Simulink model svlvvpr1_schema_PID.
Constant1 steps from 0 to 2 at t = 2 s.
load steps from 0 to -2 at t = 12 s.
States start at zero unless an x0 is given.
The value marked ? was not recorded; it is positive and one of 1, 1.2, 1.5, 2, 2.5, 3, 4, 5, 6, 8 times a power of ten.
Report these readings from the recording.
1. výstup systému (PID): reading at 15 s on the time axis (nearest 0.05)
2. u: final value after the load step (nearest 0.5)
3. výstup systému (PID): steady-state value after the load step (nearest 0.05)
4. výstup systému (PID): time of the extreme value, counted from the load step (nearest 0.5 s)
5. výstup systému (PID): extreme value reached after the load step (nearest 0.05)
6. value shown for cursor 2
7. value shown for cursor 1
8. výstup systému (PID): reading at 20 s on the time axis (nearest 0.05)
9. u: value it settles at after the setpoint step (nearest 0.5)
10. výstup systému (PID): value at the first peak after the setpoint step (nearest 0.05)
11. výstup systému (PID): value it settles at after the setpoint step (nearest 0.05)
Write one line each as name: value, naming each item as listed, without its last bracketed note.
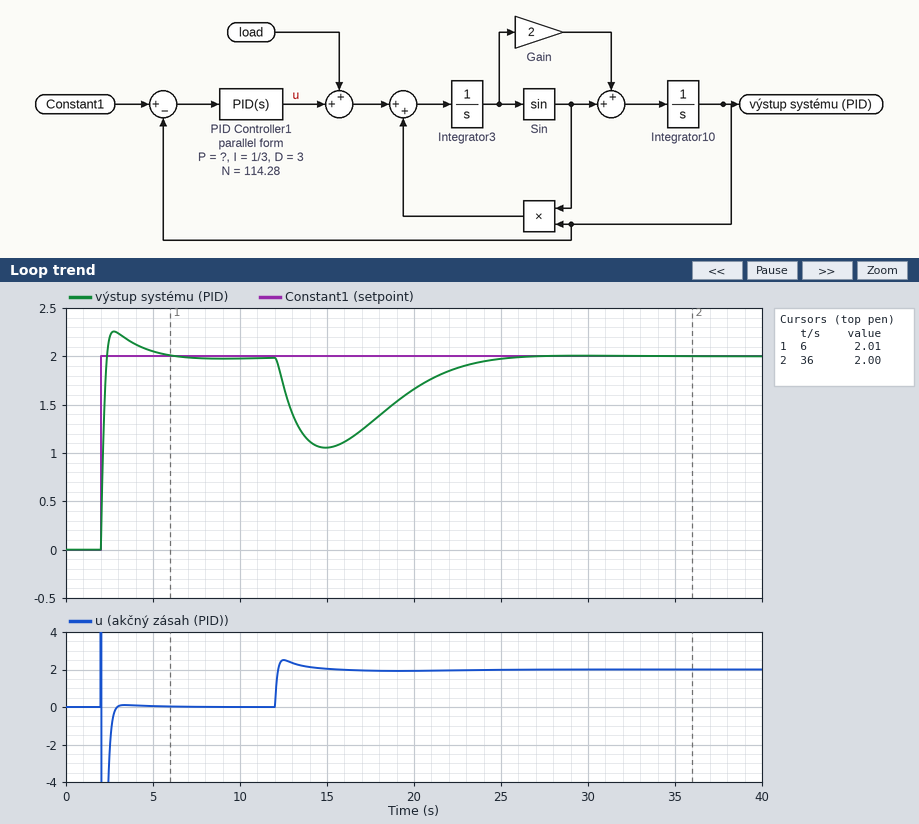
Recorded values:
výstup systému (PID): reading at 15 s on the time axis: 1.05
u: final value after the load step: 2.0
výstup systému (PID): steady-state value after the load step: 2.00
výstup systému (PID): time of the extreme value, counted from the load step: 3.0 s
výstup systému (PID): extreme value reached after the load step: 1.05
value shown for cursor 2: 2.00
value shown for cursor 1: 2.01
výstup systému (PID): reading at 20 s on the time axis: 1.65
u: value it settles at after the setpoint step: 0.0
výstup systému (PID): value at the first peak after the setpoint step: 2.25
výstup systému (PID): value it settles at after the setpoint step: 2.00
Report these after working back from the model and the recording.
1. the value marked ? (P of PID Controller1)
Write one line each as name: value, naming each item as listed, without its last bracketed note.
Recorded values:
the value marked ?: 1.5
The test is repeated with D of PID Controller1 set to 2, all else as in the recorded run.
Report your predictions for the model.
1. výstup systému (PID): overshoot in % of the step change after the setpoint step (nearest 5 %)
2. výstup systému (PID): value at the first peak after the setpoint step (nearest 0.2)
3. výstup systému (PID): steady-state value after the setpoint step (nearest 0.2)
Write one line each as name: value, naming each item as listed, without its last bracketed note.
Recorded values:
výstup systému (PID): overshoot in % of the step change after the setpoint step: 25 %
výstup systému (PID): value at the first peak after the setpoint step: 2.6
výstup systému (PID): steady-state value after the setpoint step: 2.0
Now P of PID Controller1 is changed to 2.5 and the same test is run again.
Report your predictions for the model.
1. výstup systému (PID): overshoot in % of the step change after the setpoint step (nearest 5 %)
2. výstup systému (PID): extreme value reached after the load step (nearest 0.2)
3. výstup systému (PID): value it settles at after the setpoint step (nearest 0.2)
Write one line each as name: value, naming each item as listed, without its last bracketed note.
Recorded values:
výstup systému (PID): overshoot in % of the step change after the setpoint step: 15 %
výstup systému (PID): extreme value reached after the load step: 1.4
výstup systému (PID): value it settles at after the setpoint step: 2.0
